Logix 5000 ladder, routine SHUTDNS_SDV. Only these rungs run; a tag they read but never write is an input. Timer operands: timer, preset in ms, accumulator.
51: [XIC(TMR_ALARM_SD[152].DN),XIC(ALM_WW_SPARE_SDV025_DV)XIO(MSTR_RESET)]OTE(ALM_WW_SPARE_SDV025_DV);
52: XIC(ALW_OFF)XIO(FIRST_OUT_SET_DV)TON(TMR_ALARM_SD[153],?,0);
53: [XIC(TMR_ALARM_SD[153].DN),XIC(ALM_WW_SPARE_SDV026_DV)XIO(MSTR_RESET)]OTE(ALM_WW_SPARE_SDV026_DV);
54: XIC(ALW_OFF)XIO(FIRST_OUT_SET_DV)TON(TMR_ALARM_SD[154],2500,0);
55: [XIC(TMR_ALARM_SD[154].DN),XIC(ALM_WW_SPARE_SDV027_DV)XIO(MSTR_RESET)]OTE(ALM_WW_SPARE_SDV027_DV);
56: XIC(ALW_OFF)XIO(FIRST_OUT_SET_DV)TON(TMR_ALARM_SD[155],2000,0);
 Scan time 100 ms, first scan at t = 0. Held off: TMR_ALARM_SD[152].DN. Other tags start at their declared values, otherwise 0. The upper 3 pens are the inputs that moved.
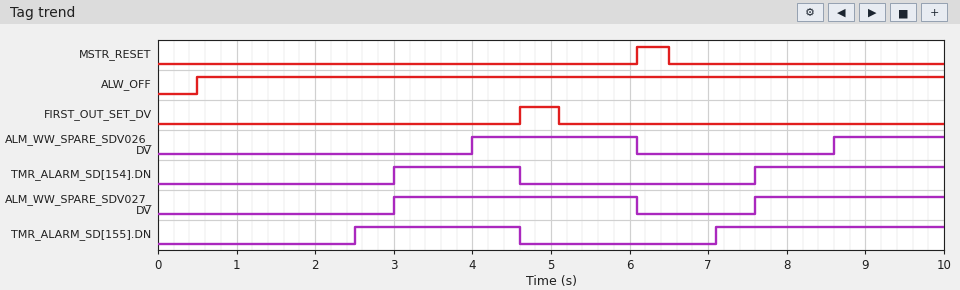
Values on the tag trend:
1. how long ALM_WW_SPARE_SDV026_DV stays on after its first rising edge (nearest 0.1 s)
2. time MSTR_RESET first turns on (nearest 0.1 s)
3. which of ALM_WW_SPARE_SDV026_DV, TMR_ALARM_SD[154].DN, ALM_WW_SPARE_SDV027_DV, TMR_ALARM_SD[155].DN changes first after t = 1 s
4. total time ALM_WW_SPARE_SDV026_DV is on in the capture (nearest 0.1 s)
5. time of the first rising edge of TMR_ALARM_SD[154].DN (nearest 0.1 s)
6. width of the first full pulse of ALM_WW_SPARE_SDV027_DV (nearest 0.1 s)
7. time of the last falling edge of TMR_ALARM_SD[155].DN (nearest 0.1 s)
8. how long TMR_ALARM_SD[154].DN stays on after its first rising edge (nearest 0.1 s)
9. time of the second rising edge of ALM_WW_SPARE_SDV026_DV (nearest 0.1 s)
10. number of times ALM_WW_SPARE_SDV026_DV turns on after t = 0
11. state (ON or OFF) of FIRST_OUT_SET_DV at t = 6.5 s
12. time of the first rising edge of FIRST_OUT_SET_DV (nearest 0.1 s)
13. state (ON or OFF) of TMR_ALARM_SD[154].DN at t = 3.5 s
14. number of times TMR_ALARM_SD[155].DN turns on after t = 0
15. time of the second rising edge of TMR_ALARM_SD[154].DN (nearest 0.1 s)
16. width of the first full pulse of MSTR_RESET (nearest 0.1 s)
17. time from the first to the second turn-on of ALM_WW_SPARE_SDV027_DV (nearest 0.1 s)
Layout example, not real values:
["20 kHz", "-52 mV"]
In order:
["2.1 s", "6.1 s", "TMR_ALARM_SD[155].DN", "3.5 s", "3.0 s", "3.1 s", "4.6 s", "1.6 s", "8.6 s", "2", "OFF", "4.6 s", "ON", "2", "7.6 s", "0.4 s", "4.6 s"]
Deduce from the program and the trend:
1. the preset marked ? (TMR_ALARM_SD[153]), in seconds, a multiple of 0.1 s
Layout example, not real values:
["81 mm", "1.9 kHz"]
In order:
["3.5 s"]
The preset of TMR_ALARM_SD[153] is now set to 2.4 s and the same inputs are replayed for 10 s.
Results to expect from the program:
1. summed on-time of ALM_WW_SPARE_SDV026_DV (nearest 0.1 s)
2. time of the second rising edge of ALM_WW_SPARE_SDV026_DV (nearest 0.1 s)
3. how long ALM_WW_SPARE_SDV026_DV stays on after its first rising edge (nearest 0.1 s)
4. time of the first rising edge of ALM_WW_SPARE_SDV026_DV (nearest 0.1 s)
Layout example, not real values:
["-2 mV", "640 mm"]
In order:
["5.7 s", "7.5 s", "3.2 s", "2.9 s"]
